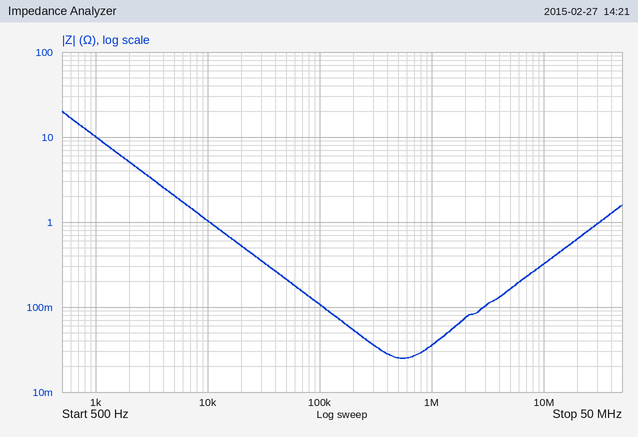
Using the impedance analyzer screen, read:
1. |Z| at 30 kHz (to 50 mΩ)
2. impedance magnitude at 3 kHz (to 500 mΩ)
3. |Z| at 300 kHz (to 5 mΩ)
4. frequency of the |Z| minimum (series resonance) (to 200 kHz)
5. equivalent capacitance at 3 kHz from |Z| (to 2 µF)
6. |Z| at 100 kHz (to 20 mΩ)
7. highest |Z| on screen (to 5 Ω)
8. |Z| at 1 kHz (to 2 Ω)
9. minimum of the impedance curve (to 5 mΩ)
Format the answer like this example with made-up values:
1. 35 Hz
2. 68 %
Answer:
1. 350 mΩ
2. 3.5 Ω
3. 35 mΩ
4. 600 kHz
5. 16 µF
6. 100 mΩ
7. 20 Ω
8. 10 Ω
9. 25 mΩ
